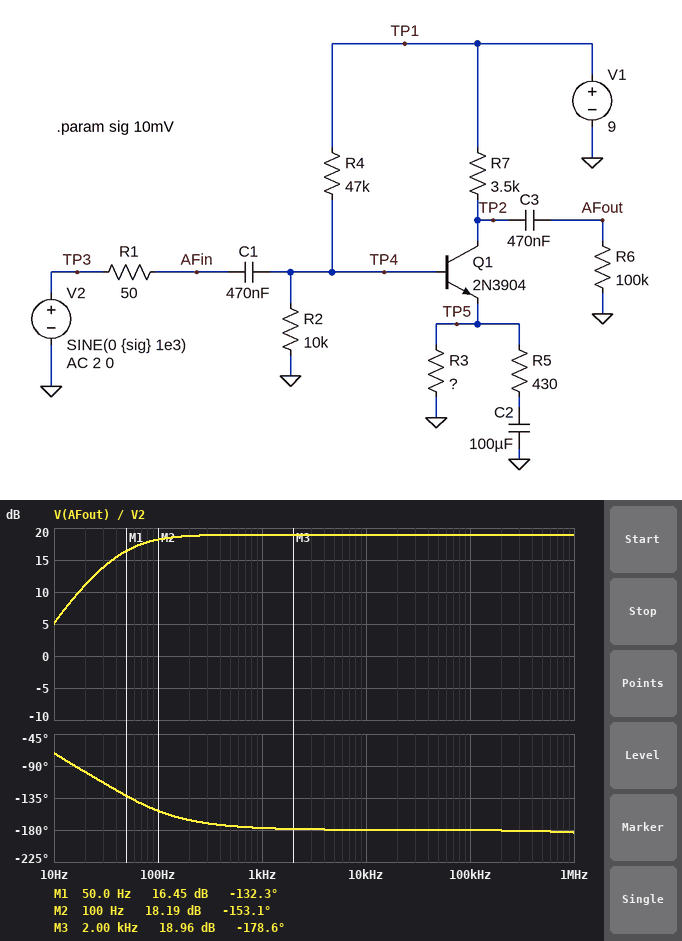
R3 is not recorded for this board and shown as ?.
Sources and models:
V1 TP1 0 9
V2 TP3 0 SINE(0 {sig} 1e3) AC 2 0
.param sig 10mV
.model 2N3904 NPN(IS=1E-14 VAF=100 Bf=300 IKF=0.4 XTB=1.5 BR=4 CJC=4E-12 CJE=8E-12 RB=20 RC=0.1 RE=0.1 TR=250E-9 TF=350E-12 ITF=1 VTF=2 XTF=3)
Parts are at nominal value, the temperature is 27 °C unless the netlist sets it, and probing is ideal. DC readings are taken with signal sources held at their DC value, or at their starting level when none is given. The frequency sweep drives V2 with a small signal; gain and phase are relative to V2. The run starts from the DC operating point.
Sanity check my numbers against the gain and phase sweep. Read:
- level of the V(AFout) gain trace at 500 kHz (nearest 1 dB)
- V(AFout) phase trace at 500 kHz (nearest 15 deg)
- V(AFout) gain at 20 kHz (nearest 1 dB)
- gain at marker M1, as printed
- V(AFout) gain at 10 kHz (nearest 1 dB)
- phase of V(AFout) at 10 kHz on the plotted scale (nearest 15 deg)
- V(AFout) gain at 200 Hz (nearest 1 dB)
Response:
19 dB
-180 deg
19 dB
16.45 dB
19 dB
-180 deg
19 dB
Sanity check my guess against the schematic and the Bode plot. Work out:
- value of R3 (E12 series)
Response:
1.5 kΩ
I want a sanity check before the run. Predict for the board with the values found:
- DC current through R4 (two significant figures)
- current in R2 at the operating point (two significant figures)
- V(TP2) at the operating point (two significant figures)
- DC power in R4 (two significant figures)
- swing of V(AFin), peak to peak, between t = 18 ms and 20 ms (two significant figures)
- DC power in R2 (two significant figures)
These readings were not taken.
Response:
160 µA
160 µA
6.9 V
1.2 mW
20 mV
240 µW
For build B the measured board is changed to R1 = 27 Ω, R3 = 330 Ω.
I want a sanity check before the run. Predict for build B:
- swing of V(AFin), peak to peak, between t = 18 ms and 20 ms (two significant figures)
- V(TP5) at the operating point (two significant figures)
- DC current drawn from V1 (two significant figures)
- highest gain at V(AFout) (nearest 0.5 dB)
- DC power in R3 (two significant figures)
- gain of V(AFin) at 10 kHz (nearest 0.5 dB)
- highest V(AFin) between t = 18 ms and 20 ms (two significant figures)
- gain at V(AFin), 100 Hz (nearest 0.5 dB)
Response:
19 mV
770 mV
2.5 mA
16.0 dB
1.8 mW
-0.5 dB
9.7 mV
0 dB
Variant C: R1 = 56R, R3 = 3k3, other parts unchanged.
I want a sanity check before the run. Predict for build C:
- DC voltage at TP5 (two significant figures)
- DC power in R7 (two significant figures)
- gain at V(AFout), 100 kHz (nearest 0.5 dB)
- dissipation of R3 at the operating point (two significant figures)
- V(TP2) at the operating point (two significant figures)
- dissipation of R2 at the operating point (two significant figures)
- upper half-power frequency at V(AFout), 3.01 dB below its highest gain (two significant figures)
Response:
950 mV
290 µW
17.0 dB
270 µW
8.0 V
250 µW
21 MHz
